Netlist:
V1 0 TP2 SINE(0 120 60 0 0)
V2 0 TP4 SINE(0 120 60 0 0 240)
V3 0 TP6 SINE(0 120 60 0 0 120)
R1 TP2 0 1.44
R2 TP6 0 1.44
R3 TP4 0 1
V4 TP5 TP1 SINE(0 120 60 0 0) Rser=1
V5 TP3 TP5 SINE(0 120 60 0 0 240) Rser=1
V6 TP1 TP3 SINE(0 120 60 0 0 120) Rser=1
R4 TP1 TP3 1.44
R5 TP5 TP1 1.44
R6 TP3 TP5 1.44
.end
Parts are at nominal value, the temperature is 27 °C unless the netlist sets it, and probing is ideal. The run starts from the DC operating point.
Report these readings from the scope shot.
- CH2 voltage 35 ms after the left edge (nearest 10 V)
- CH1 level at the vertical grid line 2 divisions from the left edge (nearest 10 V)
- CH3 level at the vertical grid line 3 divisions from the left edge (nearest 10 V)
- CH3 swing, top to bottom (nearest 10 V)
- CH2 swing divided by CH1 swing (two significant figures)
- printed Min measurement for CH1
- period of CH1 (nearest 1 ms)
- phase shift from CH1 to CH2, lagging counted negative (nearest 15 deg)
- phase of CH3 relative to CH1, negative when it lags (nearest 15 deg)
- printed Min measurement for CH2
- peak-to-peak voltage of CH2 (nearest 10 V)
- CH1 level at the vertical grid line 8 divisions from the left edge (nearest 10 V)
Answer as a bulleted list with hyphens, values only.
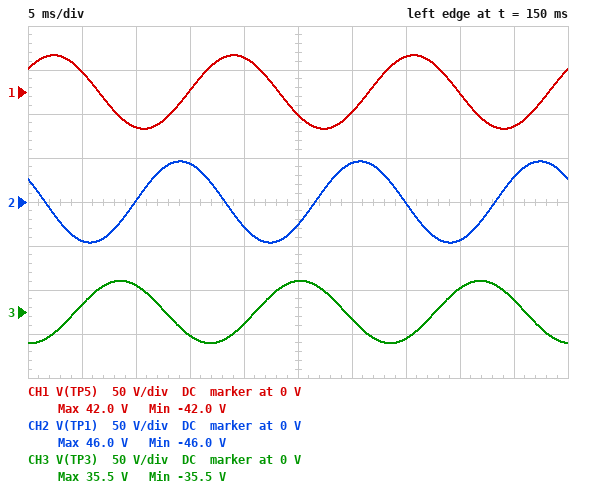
- 0 V
- -40 V
- -30 V
- 70 V
- 1.1
- -42.0 V
- 17 ms
- 105 deg
- -135 deg
- -46.0 V
- 90 V
- 0 V
